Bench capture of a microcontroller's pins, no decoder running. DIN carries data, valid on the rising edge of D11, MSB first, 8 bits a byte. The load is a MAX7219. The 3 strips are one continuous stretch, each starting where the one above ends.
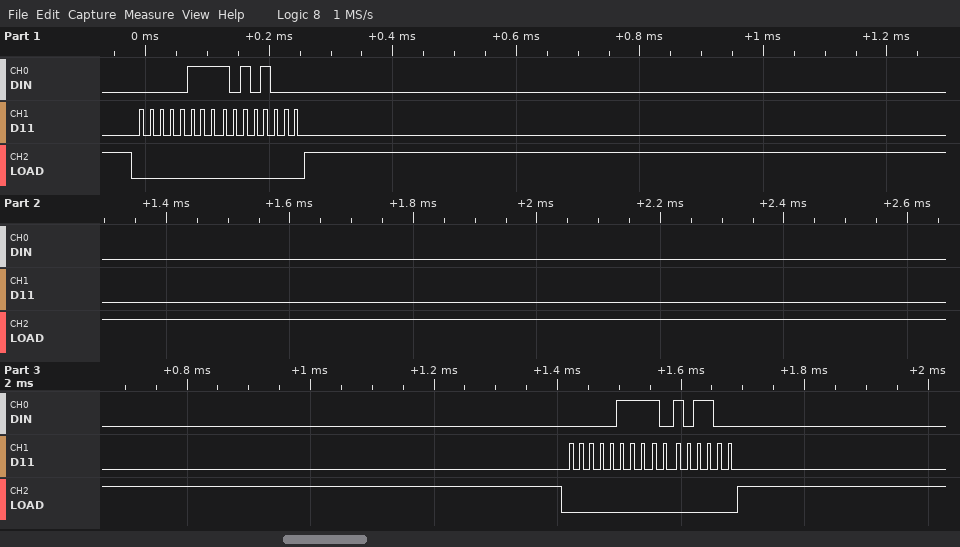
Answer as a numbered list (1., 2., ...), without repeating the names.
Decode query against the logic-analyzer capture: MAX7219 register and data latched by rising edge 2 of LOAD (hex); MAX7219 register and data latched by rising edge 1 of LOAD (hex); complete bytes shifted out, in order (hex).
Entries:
1. register 0x7, data 0xAC
2. register 0x7, data 0xA8
3. 07 A8 07 AC
